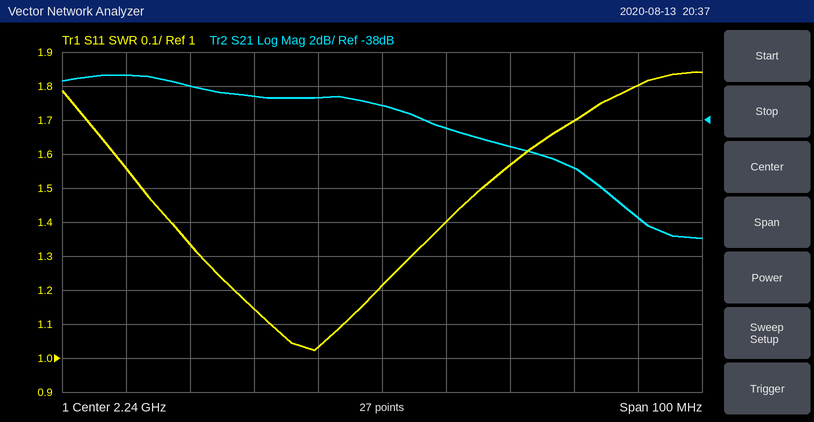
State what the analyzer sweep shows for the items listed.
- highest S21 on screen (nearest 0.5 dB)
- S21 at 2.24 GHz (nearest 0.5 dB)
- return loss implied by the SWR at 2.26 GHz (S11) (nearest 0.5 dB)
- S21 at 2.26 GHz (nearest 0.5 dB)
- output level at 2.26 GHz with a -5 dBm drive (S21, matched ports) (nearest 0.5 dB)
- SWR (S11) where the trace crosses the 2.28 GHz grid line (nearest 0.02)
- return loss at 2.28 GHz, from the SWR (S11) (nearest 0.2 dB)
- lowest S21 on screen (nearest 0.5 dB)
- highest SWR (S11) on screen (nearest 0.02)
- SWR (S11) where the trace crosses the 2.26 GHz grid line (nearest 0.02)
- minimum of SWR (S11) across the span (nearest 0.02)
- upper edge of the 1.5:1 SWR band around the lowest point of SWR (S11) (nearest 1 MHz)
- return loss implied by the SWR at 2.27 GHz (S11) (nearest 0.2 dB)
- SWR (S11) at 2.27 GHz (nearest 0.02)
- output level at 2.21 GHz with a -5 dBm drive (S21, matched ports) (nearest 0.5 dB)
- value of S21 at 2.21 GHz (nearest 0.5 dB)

-35.5 dB
-37.0 dB
13.0 dB
-39.5 dB
-44.5 dBm
1.80
10.8 dB
-45.0 dB
1.84
1.56
1.02
2.256 GHz
11.8 dB
1.70
-41.0 dBm
-36.0 dB
